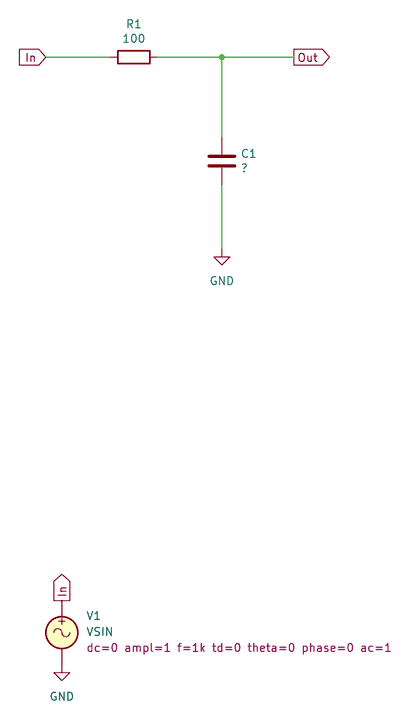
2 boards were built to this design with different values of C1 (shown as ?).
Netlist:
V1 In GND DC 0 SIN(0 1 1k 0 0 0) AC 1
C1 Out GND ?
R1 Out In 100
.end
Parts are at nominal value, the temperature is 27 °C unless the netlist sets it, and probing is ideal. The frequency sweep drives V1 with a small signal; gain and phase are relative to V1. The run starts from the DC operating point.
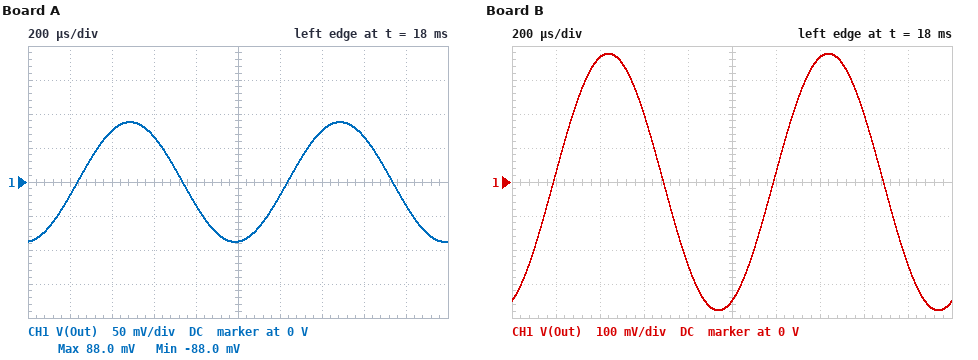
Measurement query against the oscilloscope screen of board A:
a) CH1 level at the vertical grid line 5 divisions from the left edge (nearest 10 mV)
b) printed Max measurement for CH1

-90 mV
88.0 mV
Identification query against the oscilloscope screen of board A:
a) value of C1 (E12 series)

18 µF
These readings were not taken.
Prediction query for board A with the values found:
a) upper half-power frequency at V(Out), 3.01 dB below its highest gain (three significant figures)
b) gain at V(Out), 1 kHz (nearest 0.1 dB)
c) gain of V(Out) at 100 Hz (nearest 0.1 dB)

88.4 Hz
-21.1 dB
-3.6 dB
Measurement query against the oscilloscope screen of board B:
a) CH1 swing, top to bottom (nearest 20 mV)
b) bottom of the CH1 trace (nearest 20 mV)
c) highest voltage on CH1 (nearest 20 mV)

760 mV
-380 mV
380 mV
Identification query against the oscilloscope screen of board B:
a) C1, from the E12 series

3.9 µF
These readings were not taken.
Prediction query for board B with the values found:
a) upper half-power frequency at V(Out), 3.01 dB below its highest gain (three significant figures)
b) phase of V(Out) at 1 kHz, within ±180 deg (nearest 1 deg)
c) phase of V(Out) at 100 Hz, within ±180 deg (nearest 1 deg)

408 Hz
-68 deg
-14 deg
